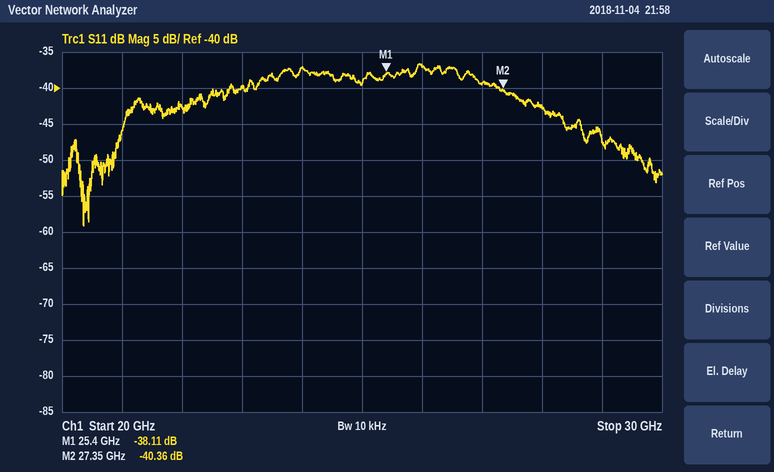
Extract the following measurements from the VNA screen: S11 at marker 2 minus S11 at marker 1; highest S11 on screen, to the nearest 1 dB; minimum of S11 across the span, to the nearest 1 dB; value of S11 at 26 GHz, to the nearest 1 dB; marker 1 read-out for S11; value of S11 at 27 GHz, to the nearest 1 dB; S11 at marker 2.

-2.25 dB
-37 dB
-59 dB
-37 dB
-38.11 dB
-39 dB
-40.36 dB
